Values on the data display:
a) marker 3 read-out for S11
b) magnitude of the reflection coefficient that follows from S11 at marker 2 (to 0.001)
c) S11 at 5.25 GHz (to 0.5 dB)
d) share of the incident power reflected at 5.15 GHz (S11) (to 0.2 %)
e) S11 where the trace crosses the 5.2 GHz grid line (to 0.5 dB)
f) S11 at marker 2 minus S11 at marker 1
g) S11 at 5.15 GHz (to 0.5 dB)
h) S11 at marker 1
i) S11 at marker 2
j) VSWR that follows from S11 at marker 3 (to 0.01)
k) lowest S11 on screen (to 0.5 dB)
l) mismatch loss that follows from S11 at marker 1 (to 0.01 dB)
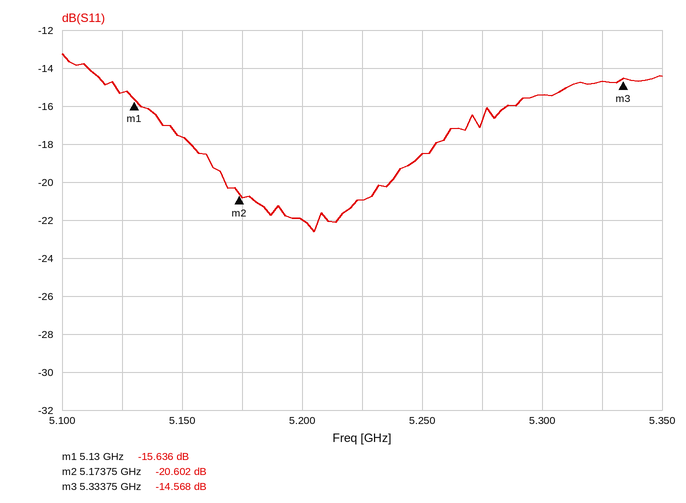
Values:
-14.568 dB
0.093
-18.5 dB
1.8 %
-22.0 dB
-4.966 dB
-17.5 dB
-15.636 dB
-20.602 dB
1.46
-22.5 dB
0.12 dB
